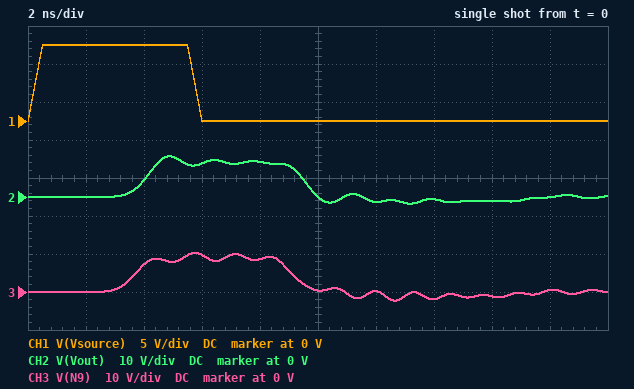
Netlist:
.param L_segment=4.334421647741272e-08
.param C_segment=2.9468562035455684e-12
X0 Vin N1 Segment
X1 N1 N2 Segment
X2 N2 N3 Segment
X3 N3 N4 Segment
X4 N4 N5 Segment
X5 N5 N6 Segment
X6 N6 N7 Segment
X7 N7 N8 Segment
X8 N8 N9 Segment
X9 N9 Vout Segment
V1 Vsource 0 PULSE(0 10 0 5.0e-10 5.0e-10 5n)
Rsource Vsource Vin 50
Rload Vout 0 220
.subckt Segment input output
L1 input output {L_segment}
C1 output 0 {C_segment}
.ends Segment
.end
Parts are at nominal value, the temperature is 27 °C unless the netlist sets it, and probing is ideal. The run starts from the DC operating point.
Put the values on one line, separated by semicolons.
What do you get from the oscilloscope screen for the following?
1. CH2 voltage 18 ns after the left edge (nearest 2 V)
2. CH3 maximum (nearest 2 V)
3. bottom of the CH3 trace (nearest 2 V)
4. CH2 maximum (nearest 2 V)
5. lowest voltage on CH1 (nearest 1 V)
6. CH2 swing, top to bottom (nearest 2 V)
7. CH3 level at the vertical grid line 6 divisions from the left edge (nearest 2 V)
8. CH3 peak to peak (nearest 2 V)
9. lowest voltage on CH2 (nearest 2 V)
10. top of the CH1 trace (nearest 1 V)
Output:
0 V; 10 V; -2 V; 10 V; 0 V; 12 V; 0 V; 12 V; -2 V; 10 V
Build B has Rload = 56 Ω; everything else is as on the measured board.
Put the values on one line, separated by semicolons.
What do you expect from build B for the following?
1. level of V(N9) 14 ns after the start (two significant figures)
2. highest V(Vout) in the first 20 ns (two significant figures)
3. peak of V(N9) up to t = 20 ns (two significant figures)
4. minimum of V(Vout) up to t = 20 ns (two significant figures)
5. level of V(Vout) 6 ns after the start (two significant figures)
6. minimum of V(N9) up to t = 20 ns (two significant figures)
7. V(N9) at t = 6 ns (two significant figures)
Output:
320 mV; 5.2 V; 7.0 V; -670 mV; 4.4 V; -2.2 V; 5.5 V
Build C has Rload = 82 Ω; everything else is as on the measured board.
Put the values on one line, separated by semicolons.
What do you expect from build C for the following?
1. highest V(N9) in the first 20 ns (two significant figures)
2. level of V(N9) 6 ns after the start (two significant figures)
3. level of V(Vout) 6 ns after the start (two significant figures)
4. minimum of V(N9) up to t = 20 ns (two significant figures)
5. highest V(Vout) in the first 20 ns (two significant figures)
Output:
7.5 V; 6.6 V; 5.6 V; -1.4 V; 6.7 V
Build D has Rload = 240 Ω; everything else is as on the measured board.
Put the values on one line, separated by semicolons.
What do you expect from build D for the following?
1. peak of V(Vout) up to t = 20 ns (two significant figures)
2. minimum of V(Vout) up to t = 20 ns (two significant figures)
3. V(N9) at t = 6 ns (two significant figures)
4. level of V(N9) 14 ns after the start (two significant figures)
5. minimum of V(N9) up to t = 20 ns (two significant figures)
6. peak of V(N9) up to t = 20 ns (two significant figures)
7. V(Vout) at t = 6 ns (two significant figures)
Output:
11 V; -2.0 V; 10 V; -2.1 V; -2.5 V; 11 V; 9.1 V
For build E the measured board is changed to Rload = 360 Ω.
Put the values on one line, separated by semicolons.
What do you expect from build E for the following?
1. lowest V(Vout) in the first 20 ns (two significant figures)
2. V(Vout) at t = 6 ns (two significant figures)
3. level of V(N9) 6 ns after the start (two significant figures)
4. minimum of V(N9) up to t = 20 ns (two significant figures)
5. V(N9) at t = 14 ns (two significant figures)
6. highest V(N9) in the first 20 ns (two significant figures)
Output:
-3.0 V; 10 V; 11 V; -3.5 V; -3.1 V; 12 V
